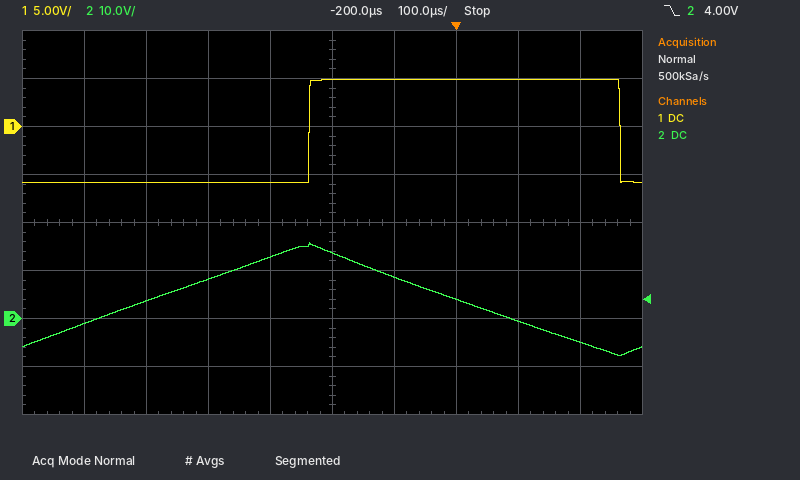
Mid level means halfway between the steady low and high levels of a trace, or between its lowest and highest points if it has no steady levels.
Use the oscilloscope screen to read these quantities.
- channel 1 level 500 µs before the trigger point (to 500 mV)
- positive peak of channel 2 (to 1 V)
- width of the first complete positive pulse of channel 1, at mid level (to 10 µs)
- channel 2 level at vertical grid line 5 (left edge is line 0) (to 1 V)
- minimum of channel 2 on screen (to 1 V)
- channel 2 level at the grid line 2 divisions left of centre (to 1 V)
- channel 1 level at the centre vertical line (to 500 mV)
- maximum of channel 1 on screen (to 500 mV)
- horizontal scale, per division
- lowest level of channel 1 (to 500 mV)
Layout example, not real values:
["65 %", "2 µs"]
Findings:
["-6.0 V", "16 V", "500 µs", "14 V", "-8 V", "8 V", "5.0 V", "5.0 V", "100 µs", "-6.0 V"]
